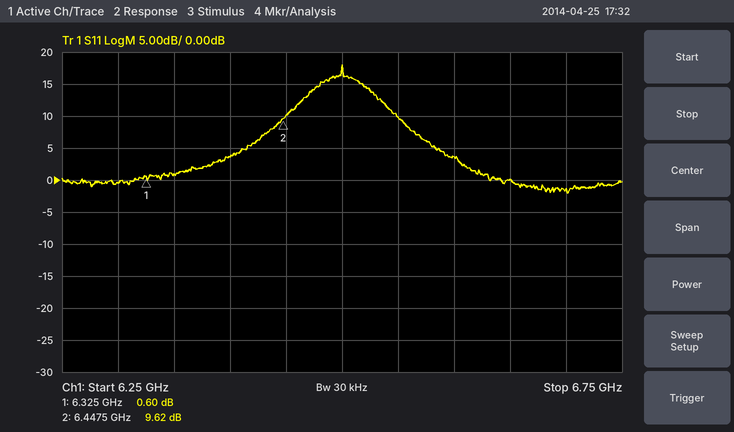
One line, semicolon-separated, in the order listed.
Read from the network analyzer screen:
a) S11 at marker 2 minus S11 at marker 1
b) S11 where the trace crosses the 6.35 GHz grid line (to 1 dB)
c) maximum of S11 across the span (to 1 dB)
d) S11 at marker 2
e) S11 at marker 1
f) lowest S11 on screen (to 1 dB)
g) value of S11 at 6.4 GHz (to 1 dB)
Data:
9.02 dB; 1 dB; 18 dB; 9.62 dB; 0.60 dB; -2 dB; 4 dB
